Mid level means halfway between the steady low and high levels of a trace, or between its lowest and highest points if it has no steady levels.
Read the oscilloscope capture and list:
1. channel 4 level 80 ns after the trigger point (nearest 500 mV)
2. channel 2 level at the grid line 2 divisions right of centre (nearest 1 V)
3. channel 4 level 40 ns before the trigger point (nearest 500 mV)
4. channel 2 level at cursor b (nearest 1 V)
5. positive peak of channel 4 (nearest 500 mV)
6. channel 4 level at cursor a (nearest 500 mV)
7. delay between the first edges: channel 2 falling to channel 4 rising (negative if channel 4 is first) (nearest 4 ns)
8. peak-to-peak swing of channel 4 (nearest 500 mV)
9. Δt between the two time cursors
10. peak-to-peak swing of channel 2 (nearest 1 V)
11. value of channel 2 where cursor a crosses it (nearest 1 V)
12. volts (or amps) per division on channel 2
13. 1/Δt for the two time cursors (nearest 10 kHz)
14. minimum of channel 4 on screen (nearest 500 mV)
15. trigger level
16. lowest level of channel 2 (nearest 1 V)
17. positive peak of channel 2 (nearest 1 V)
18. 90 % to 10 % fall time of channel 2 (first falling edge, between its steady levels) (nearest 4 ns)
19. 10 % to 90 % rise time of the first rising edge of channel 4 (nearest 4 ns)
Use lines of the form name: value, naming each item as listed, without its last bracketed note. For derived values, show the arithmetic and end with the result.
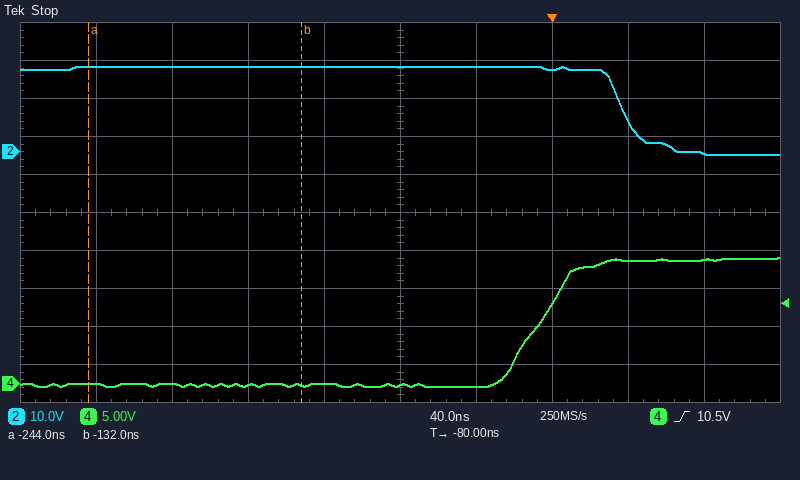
channel 4 level 80 ns after the trigger point: 16.5 V
channel 2 level at the grid line 2 divisions right of centre: 22 V
channel 4 level 40 ns before the trigger point: -500 mV
channel 2 level at cursor b: 22 V
positive peak of channel 4: 16.5 V
channel 4 level at cursor a: 0.0 V
delay between the first edges: channel 2 falling to channel 4 rising (negative if channel 4 is first): -44 ns
peak-to-peak swing of channel 4: 16.5 V − (-500 mV) = 17.0 V
Δt between the two time cursors: -132 ns − (-244 ns) = 112 ns
peak-to-peak swing of channel 2: 22 V − (-1 V) = 23 V
value of channel 2 where cursor a crosses it: 22 V
volts (or amps) per division on channel 2: 10 V
1/Δt for the two time cursors: 1 / 112 ns ≈ 8.93 MHz
minimum of channel 4 on screen: -500 mV
trigger level: 10.5 V
lowest level of channel 2: -1 V
positive peak of channel 2: 22 V
90 % to 10 % fall time of channel 2 (first falling edge, between its steady levels): 32 ns
10 % to 90 % rise time of the first rising edge of channel 4: 32 ns
